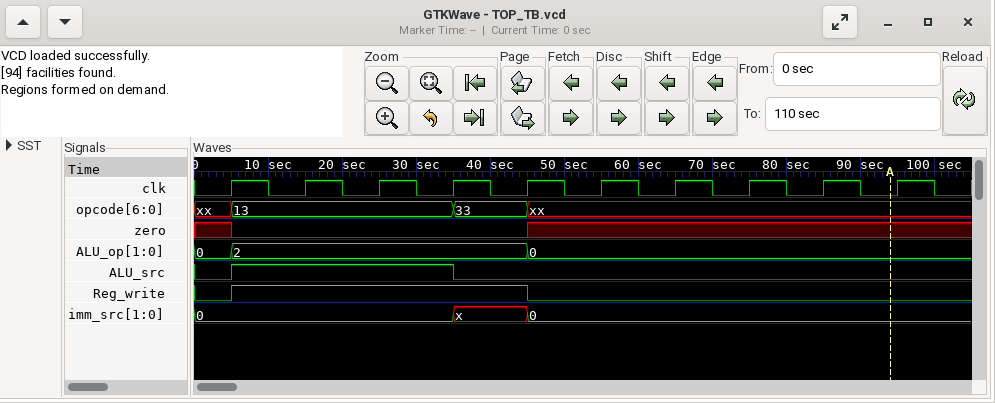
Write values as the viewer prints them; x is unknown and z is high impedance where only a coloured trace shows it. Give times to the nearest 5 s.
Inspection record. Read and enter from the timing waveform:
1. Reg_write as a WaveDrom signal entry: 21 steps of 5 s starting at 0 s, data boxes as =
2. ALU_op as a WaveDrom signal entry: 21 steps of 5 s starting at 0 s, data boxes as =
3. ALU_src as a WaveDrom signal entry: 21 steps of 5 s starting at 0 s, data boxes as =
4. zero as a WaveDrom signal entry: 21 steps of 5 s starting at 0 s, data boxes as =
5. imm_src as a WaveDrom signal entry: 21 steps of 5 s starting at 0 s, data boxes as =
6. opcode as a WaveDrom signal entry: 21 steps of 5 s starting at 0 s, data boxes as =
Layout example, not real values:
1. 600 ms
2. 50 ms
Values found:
1. {name: 'Reg_write', wave: '01.......0...........'}
2. {name: 'ALU_op', wave: '==.......=...........', data: '0 2 0'}
3. {name: 'ALU_src', wave: '01.....0.............'}
4. {name: 'zero', wave: 'x0.......x...........'}
5. {name: 'imm_src', wave: '=......x.=...........', data: '0 0'}
6. {name: 'opcode', wave: 'x=.....=.x...........', data: '13 33'}
